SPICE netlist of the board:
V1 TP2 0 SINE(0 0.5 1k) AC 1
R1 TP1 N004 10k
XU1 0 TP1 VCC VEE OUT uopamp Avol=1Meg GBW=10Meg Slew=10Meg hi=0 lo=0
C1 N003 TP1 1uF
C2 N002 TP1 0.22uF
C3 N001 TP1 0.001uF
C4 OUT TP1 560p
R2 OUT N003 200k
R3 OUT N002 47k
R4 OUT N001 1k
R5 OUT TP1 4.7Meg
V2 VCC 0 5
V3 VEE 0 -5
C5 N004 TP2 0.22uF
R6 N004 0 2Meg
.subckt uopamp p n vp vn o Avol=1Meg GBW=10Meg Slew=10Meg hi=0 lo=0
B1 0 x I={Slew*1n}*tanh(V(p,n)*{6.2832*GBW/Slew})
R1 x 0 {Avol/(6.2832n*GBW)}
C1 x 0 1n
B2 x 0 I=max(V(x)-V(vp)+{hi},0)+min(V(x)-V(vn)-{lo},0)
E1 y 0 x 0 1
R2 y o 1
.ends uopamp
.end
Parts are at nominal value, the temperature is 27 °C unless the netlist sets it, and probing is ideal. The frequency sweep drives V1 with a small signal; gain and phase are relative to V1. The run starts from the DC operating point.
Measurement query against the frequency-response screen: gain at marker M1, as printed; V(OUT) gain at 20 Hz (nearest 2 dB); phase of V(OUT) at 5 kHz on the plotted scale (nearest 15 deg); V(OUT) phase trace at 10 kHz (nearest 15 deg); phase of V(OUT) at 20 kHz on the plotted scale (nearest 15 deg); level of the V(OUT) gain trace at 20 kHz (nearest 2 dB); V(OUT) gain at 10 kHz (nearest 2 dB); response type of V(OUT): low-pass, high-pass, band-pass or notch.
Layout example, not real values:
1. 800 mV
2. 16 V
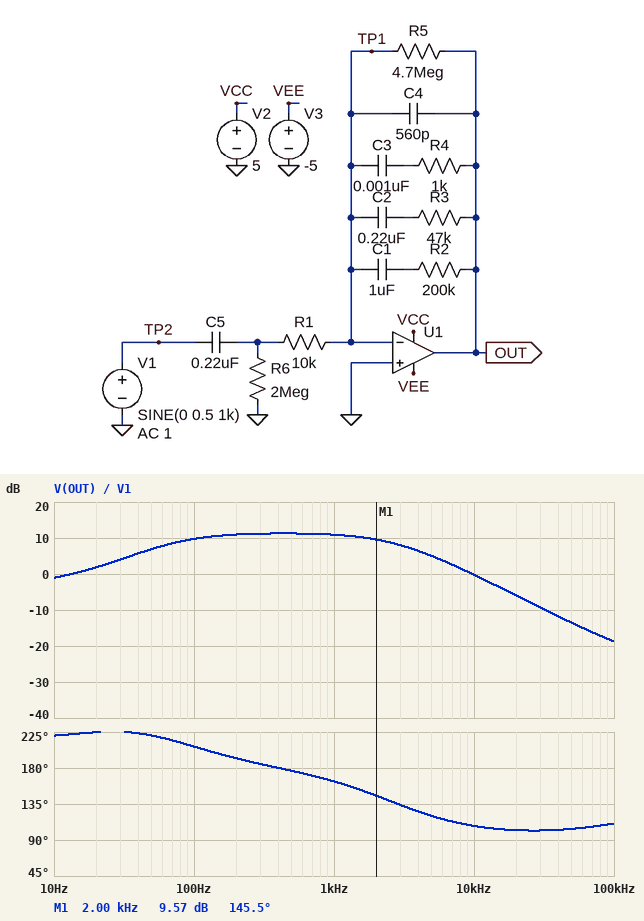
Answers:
1. 9.57 dB
2. 2 dB
3. 120 deg
4. 105 deg
5. 105 deg
6. -6 dB
7. 0 dB
8. band-pass
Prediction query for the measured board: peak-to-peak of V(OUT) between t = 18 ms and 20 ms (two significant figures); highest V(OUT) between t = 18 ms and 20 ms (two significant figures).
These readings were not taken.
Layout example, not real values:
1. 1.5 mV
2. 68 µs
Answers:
1. 3.5 V
2. 1.8 V
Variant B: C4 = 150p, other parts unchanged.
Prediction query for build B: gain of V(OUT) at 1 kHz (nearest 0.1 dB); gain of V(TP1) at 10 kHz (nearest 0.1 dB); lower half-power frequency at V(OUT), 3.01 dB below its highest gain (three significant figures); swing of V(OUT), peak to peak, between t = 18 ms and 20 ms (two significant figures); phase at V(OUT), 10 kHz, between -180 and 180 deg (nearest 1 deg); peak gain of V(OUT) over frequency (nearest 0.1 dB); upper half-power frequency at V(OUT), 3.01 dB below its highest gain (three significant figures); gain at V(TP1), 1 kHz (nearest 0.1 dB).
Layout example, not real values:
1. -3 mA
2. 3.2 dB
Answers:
1. 11.2 dB
2. -57.9 dB
3. 66.8 Hz
4. 3.6 V
5. 113 deg
6. 11.3 dB
7. 3.74 kHz
8. -68.8 dB
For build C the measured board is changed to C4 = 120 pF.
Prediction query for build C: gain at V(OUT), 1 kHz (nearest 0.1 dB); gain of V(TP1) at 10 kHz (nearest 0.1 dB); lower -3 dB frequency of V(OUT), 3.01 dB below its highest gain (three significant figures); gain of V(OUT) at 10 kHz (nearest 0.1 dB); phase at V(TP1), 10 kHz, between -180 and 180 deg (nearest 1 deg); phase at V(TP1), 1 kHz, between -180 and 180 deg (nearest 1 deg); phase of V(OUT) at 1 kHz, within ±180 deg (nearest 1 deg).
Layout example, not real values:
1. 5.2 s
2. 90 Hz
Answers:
1. 11.2 dB
2. -57.7 dB
3. 66.9 Hz
4. 2.3 dB
5. 24 deg
6. 78 deg
7. 169 deg
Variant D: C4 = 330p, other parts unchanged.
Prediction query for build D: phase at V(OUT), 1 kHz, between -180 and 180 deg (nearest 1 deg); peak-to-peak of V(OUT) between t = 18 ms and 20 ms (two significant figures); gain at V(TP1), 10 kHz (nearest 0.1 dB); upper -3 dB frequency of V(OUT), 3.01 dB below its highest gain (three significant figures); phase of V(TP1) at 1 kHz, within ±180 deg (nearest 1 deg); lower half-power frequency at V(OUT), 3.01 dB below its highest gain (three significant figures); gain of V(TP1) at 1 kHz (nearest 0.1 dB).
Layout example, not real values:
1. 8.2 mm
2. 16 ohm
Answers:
1. 166 deg
2. 3.6 V
3. -59.0 dB
4. 3.27 kHz
5. 75 deg
6. 66.5 Hz
7. -68.9 dB
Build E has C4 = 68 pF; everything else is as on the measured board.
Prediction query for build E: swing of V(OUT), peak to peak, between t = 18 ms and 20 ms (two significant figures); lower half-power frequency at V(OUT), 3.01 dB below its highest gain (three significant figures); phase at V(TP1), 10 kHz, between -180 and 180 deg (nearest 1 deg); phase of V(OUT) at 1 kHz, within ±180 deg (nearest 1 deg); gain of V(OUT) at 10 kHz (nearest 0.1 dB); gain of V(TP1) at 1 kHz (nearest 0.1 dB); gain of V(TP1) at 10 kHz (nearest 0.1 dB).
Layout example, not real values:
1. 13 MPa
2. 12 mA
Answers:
1. 3.6 V
2. 67.0 Hz
3. 25 deg
4. 169 deg
5. 2.7 dB
6. -68.8 dB
7. -57.3 dB
